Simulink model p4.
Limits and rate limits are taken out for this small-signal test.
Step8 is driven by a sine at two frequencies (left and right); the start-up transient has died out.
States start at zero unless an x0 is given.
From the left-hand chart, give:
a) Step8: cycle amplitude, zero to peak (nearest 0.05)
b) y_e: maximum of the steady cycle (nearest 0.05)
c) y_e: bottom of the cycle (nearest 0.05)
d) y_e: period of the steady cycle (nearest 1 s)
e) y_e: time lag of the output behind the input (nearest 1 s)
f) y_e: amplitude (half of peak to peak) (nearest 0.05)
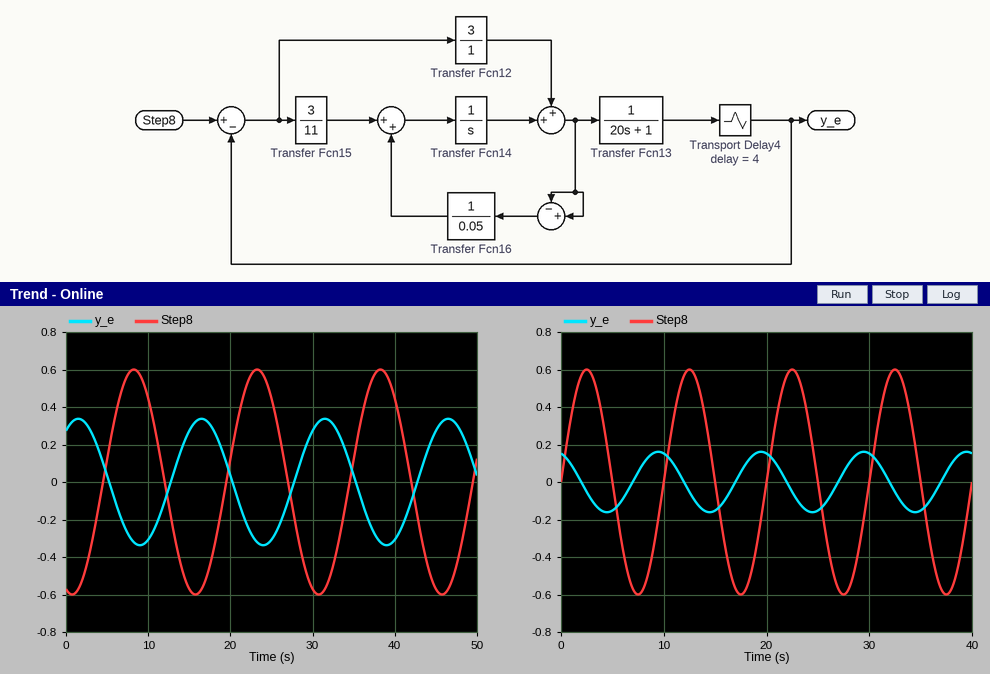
0.60
0.35
-0.35
15 s
8 s
0.35
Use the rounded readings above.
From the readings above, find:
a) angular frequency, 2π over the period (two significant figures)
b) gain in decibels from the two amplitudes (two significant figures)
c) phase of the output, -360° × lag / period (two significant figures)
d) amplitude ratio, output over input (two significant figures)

0.42 rad/s
-4.7 dB
-190°
0.58
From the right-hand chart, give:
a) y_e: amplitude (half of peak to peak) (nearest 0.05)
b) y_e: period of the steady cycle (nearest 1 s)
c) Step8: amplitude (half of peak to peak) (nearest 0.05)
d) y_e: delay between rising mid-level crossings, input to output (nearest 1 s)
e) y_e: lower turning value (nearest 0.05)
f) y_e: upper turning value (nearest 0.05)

0.15
10 s
0.60
7 s
-0.15
0.15
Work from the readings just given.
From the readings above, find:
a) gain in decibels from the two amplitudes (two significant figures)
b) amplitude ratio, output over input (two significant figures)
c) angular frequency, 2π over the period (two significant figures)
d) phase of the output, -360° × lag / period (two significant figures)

-12 dB
0.25
0.63 rad/s
-250°
